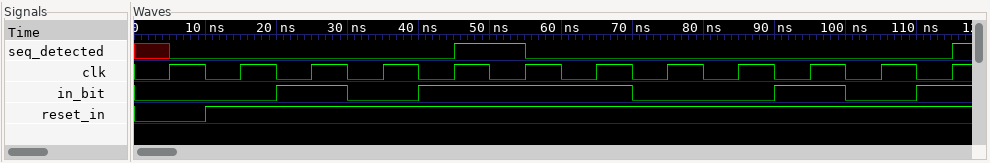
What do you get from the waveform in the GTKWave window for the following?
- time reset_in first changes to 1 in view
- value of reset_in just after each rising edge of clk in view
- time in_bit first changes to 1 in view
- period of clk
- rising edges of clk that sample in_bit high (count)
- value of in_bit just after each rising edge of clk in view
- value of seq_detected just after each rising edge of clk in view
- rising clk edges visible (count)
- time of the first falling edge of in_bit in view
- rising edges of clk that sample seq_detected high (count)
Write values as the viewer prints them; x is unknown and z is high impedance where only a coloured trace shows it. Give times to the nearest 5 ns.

10 ns
0 1 1 1 1 1 1 1 1 1 1 1
20 ns
10 ns
6
0 0 1 0 1 1 1 0 0 1 0 1
0 0 0 0 1 0 0 0 0 0 0 1
12
30 ns
1
